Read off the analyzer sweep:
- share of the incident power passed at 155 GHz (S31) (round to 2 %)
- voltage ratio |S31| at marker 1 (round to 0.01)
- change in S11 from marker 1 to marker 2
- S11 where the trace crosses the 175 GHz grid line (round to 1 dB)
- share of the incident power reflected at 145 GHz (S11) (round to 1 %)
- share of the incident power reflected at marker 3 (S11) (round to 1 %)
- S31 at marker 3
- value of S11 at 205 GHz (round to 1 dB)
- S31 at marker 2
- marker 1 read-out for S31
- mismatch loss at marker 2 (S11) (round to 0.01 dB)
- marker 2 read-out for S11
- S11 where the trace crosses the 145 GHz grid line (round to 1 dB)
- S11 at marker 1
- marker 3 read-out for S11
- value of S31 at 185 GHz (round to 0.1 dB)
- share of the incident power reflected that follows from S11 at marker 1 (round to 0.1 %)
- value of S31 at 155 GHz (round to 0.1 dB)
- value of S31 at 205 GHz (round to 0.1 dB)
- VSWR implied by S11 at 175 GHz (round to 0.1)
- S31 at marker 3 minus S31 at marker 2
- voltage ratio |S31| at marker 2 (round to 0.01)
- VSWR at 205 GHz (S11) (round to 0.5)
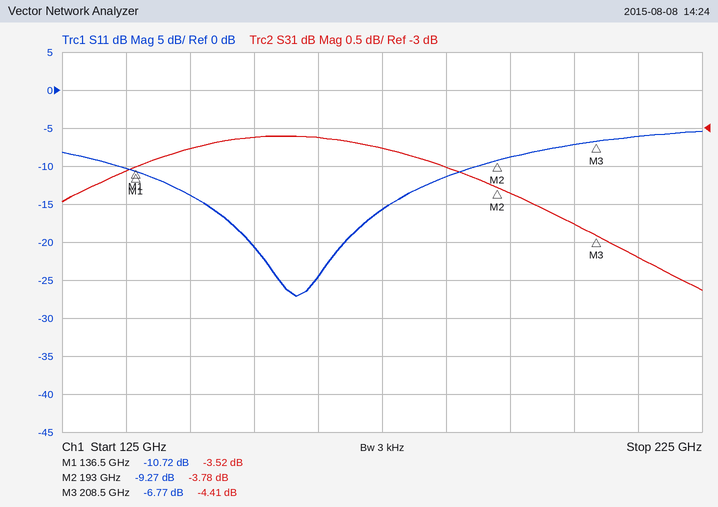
48 %
0.67
1.45 dB
-16 dB
4 %
21 %
-4.41 dB
-7 dB
-3.78 dB
-3.52 dB
0.55 dB
-9.27 dB
-14 dB
-10.72 dB
-6.77 dB
-3.5 dB
8.5 %
-3.1 dB
-4.3 dB
1.4
-0.63 dB
0.65
2.5
